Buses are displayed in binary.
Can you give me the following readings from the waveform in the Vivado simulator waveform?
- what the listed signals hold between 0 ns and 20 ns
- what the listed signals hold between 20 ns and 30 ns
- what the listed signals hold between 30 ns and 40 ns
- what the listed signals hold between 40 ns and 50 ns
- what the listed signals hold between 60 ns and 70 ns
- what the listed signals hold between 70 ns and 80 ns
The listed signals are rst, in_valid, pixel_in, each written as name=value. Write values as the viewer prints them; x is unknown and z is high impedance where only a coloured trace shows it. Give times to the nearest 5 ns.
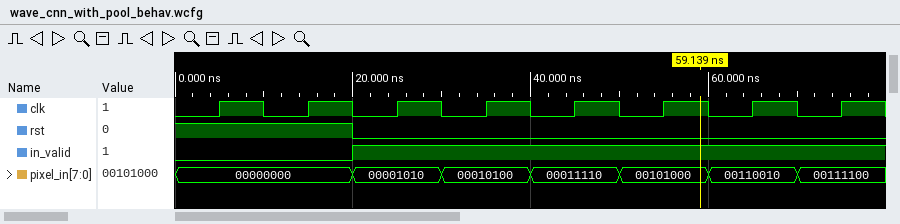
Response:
rst=1, in_valid=0, pixel_in=00000000
rst=0, in_valid=1, pixel_in=00001010
rst=0, in_valid=1, pixel_in=00010100
rst=0, in_valid=1, pixel_in=00011110
rst=0, in_valid=1, pixel_in=00110010
rst=0, in_valid=1, pixel_in=00111100
